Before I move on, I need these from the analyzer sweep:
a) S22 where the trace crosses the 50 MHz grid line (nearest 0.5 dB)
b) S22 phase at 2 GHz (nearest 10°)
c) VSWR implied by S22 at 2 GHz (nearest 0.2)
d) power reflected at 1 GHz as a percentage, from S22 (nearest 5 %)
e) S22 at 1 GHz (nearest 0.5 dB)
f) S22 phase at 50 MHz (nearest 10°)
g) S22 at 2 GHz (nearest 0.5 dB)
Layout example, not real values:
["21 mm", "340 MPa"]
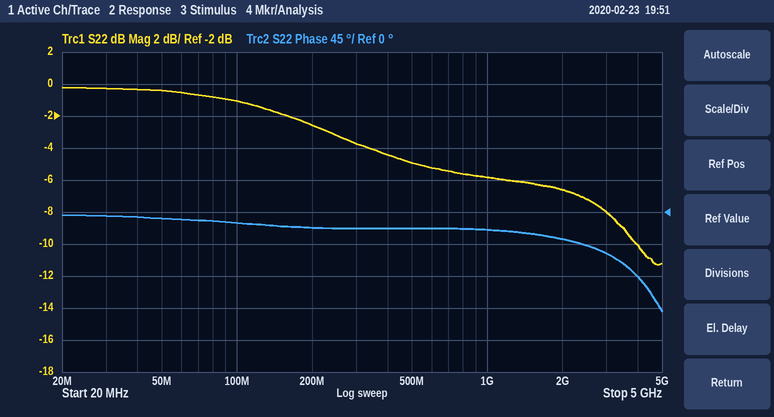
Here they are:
["-0.5 dB", "-40°", "2.8", "25 %", "-6.0 dB", "-10°", "-6.5 dB"]
